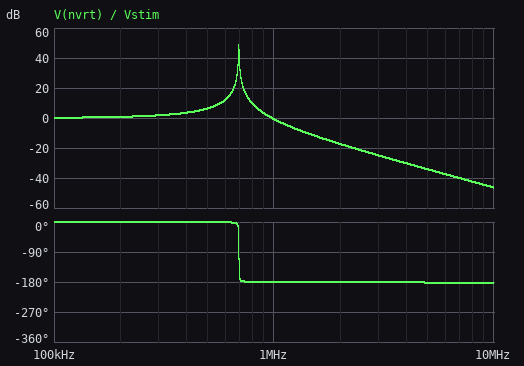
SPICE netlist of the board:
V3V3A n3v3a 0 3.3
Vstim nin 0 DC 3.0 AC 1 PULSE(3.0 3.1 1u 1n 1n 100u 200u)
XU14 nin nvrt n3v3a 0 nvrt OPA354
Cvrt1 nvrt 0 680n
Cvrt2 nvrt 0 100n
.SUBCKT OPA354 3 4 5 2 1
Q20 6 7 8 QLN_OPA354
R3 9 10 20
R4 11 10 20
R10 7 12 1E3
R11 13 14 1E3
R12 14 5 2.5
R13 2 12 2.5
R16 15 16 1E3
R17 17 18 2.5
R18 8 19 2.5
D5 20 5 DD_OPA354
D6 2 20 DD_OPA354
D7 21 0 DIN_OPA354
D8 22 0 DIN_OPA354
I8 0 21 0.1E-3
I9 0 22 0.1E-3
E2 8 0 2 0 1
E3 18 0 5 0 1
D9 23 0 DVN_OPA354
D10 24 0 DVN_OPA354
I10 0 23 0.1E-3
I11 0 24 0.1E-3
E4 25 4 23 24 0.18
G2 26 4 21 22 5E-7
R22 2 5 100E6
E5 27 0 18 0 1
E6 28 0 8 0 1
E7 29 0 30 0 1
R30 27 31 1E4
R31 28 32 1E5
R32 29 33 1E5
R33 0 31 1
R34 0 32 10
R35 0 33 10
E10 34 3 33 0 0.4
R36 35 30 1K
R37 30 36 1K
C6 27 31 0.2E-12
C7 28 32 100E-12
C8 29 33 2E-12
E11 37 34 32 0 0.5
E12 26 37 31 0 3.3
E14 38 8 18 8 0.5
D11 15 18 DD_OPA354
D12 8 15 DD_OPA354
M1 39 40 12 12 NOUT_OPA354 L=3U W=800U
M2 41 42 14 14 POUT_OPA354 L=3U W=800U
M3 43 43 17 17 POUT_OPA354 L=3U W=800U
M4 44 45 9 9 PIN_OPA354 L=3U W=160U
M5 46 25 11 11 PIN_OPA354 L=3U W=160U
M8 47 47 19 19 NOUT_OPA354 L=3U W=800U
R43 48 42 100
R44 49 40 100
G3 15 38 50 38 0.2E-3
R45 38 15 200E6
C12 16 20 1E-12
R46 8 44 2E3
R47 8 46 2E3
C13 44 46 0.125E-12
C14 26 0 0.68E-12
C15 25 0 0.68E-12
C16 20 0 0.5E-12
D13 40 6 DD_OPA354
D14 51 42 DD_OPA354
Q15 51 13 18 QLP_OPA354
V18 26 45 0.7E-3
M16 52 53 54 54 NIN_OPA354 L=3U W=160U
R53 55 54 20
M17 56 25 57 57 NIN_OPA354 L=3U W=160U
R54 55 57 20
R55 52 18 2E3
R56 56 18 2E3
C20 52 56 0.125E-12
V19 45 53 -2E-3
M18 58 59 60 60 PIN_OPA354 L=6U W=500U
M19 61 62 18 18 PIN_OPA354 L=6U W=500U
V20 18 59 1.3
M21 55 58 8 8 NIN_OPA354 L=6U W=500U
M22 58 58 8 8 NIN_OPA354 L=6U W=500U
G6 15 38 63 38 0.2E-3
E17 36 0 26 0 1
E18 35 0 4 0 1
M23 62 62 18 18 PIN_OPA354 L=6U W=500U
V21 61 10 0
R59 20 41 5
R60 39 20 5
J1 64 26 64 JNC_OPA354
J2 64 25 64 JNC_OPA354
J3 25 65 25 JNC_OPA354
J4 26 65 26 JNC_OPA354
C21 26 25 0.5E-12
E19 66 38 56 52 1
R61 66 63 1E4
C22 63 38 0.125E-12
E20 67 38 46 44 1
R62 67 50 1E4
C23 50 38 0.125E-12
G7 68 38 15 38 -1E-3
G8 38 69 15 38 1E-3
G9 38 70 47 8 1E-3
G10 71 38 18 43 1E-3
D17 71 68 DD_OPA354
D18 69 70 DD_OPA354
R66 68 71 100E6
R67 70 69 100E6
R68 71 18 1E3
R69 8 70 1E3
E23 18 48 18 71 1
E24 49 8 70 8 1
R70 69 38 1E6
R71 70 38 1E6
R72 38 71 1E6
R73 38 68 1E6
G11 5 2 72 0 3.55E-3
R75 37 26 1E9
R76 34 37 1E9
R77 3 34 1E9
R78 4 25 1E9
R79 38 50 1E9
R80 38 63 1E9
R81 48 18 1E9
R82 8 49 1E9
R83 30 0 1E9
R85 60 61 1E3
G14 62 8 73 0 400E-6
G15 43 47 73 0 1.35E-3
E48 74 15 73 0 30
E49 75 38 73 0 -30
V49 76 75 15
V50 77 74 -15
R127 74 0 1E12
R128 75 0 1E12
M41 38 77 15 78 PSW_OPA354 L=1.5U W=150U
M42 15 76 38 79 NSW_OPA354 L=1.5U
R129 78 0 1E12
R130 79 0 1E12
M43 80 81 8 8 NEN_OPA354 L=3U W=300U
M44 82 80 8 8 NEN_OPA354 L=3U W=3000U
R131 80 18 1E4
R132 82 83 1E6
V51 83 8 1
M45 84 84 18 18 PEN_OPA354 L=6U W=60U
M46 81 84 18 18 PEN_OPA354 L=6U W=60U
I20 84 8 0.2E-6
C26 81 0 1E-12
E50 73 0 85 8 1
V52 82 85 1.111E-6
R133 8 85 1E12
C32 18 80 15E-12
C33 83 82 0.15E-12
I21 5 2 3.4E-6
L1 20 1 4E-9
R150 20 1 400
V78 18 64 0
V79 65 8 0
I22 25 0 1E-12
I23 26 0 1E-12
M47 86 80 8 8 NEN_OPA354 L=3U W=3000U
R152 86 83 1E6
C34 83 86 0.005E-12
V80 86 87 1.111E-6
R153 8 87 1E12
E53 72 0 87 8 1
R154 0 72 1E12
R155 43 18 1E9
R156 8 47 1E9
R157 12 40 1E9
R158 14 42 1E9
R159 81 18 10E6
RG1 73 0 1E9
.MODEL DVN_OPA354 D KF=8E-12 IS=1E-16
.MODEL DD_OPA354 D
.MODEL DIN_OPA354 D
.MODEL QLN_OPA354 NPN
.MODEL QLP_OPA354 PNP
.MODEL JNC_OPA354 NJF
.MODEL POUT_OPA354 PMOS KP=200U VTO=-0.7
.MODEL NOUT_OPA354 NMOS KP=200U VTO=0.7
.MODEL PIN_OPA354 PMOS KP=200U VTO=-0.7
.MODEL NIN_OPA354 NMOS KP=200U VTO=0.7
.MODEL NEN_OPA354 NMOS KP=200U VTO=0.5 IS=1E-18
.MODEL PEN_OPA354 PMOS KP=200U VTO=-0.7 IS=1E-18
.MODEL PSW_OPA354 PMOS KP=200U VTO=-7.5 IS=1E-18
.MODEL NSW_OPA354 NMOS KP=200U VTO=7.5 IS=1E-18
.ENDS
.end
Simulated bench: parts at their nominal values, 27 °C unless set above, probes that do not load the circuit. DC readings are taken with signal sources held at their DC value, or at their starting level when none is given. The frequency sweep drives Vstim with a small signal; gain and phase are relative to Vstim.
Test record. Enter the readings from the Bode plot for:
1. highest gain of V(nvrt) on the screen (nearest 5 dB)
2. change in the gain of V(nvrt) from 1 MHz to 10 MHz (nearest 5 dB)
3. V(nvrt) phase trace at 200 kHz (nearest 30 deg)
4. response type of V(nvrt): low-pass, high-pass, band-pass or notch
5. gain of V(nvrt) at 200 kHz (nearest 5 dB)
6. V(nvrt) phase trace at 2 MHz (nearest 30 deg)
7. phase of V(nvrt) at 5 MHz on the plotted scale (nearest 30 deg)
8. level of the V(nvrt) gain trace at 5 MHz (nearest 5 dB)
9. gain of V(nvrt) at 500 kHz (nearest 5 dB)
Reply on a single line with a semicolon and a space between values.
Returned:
50 dB; -45 dB; 0 deg; low-pass; 0 dB; -180 deg; -180 deg; -35 dB; 5 dB
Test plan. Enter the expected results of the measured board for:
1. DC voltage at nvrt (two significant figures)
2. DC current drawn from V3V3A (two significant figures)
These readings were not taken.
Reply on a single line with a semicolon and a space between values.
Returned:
3.0 V; 4.9 mA
